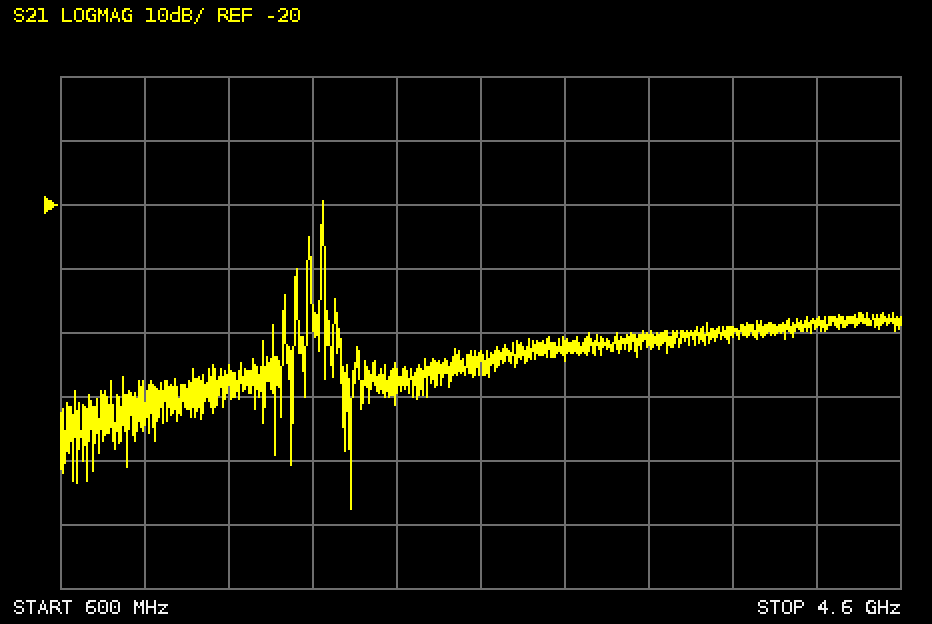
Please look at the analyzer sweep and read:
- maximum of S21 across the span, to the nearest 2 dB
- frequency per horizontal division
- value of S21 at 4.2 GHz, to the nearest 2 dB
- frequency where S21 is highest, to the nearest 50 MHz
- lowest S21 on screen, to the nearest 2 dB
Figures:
-20 dB
400 MHz
-38 dB
1.85 GHz
-68 dB
